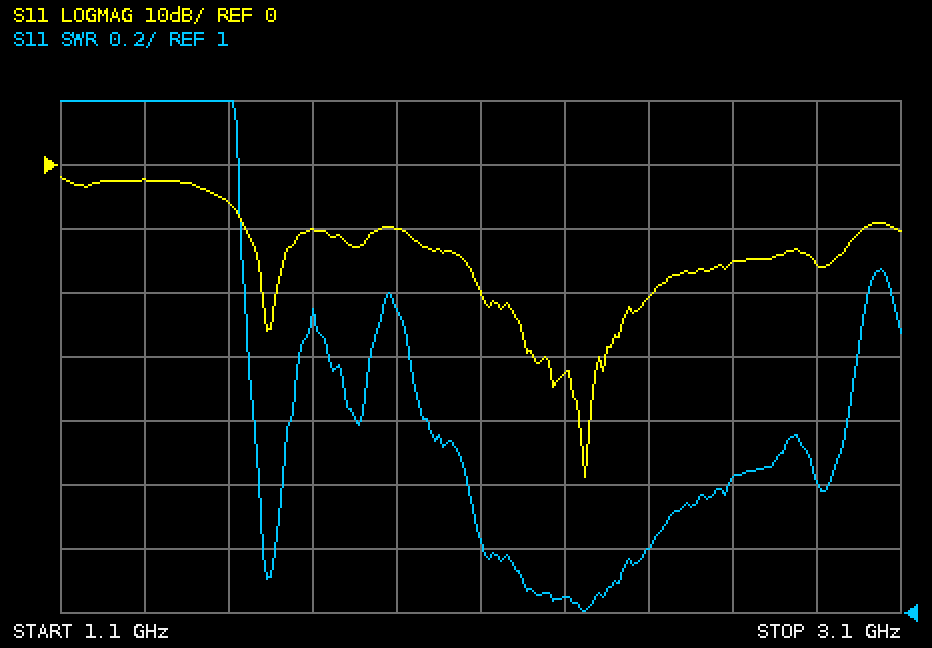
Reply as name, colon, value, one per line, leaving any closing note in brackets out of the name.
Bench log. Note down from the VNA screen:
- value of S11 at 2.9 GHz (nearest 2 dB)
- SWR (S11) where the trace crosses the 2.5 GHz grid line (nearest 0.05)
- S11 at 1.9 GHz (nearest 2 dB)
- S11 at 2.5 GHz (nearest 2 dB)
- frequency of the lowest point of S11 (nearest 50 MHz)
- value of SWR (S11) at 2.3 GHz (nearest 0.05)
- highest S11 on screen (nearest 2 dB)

value of S11 at 2.9 GHz: -16 dB
SWR (S11) where the trace crosses the 2.5 GHz grid line: 1.20
S11 at 1.9 GHz: -10 dB
S11 at 2.5 GHz: -20 dB
frequency of the lowest point of S11: 2.35 GHz
value of SWR (S11) at 2.3 GHz: 1.05
highest S11 on screen: -2 dB
